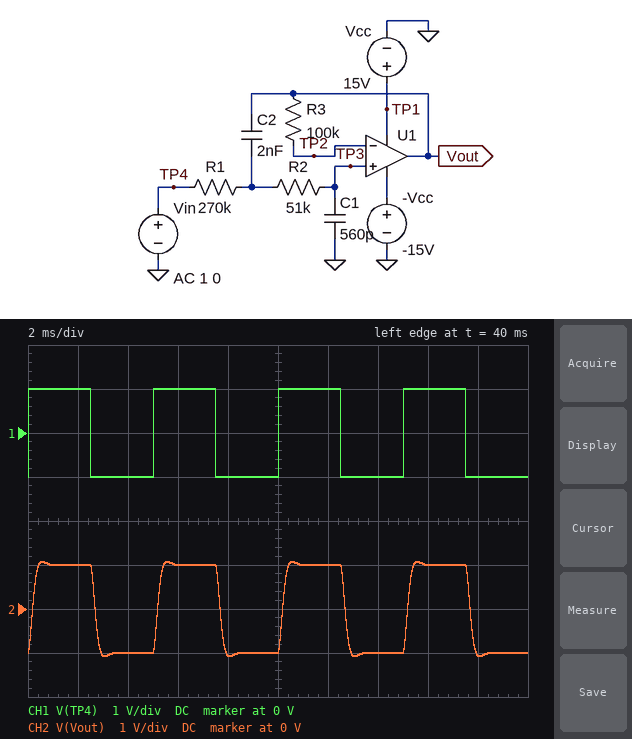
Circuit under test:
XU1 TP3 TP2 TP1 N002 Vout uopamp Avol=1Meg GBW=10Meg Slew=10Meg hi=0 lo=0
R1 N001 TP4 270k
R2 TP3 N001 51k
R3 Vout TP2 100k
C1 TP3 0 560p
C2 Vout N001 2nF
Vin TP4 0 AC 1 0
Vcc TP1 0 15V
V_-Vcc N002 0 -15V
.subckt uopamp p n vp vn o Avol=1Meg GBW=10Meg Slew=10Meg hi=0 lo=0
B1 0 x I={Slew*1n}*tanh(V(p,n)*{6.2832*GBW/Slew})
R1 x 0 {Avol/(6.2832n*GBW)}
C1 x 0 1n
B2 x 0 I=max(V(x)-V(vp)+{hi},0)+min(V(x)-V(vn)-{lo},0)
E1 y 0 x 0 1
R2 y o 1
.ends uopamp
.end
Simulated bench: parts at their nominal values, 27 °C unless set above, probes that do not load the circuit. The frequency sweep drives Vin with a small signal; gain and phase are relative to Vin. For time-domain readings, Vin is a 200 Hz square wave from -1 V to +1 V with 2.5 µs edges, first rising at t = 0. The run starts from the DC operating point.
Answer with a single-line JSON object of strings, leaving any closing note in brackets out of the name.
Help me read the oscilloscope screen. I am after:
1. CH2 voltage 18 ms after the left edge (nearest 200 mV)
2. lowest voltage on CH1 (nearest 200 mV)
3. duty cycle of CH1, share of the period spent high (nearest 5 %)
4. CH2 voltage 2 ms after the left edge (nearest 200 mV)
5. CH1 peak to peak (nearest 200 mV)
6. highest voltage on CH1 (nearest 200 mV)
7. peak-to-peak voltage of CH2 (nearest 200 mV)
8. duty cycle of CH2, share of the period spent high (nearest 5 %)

{"CH2 voltage 18 ms after the left edge": "-1.0 V", "lowest voltage on CH1": "-1.0 V", "duty cycle of CH1, share of the period spent high": "50 %", "CH2 voltage 2 ms after the left edge": "1.0 V", "CH1 peak to peak": "2.0 V", "highest voltage on CH1": "1.0 V", "peak-to-peak voltage of CH2": "2.2 V", "duty cycle of CH2, share of the period spent high": "50 %"}
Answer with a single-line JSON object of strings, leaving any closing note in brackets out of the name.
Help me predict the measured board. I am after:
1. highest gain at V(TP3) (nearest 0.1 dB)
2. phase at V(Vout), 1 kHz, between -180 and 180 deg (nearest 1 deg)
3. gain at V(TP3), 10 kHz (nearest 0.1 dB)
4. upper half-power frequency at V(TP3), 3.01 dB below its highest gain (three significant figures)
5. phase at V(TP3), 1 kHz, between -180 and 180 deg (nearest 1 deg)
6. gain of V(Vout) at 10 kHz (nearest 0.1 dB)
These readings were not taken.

{"highest gain at V(TP3)": "0 dB", "phase at V(Vout), 1 kHz, between -180 and 180 deg": "-71 deg", "gain at V(TP3), 10 kHz": "-35.7 dB", "upper half-power frequency at V(TP3), 3.01 dB below its highest gain": "1.25 kHz", "phase at V(TP3), 1 kHz, between -180 and 180 deg": "-71 deg", "gain of V(Vout) at 10 kHz": "-35.7 dB"}
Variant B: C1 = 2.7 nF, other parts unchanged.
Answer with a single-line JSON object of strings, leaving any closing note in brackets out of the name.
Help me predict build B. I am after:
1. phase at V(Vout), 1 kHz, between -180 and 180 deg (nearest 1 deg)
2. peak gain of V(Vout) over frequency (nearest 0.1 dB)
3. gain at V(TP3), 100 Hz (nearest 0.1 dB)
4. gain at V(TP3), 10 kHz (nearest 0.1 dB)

{"phase at V(Vout), 1 kHz, between -180 and 180 deg": "-110 deg", "peak gain of V(Vout) over frequency": "0 dB", "gain at V(TP3), 100 Hz": "-0.9 dB", "gain at V(TP3), 10 kHz": "-49.5 dB"}
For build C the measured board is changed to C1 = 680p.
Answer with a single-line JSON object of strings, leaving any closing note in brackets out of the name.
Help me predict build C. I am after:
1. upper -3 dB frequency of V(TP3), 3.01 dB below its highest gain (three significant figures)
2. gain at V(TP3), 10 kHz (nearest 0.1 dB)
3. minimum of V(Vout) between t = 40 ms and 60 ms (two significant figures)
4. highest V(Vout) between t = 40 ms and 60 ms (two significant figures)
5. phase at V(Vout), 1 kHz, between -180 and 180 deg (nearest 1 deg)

{"upper -3 dB frequency of V(TP3), 3.01 dB below its highest gain": "1.02 kHz", "gain at V(TP3), 10 kHz": "-37.4 dB", "minimum of V(Vout) between t = 40 ms and 60 ms": "-1.0 V", "highest V(Vout) between t = 40 ms and 60 ms": "1.0 V", "phase at V(Vout), 1 kHz, between -180 and 180 deg": "-79 deg"}
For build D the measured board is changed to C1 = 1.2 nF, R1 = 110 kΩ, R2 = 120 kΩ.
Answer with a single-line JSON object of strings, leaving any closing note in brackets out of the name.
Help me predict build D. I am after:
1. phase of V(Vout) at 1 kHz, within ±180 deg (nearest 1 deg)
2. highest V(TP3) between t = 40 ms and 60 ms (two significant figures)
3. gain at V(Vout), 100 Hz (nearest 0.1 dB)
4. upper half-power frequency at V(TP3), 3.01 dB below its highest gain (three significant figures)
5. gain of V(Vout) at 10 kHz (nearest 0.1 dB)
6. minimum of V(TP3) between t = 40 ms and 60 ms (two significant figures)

{"phase of V(Vout) at 1 kHz, within ±180 deg": "-98 deg", "highest V(TP3) between t = 40 ms and 60 ms": "1.0 V", "gain at V(Vout), 100 Hz": "0 dB", "upper half-power frequency at V(TP3), 3.01 dB below its highest gain": "809 Hz", "gain of V(Vout) at 10 kHz": "-42.0 dB", "minimum of V(TP3) between t = 40 ms and 60 ms": "-1.0 V"}
